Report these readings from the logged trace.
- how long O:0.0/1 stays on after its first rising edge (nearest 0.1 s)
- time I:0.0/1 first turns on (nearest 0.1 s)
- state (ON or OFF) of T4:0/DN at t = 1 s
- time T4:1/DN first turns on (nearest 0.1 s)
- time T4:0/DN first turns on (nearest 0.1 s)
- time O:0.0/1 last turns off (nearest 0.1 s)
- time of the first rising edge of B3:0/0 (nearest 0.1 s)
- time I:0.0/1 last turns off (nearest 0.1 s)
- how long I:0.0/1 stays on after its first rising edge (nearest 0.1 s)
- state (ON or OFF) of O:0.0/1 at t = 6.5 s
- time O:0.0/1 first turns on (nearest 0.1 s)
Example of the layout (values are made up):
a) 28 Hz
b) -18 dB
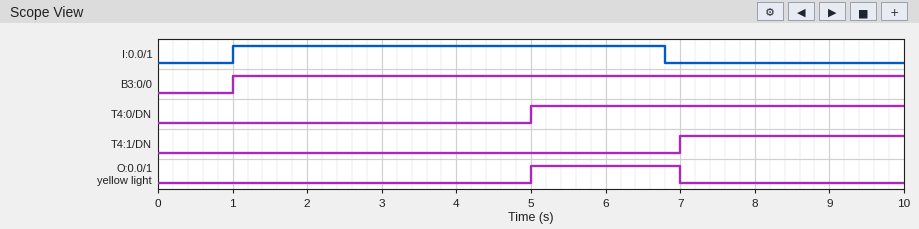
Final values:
a) 2.0 s
b) 1.0 s
c) OFF
d) 7.0 s
e) 5.0 s
f) 7.0 s
g) 1.0 s
h) 6.8 s
i) 5.8 s
j) ON
k) 5.0 s
